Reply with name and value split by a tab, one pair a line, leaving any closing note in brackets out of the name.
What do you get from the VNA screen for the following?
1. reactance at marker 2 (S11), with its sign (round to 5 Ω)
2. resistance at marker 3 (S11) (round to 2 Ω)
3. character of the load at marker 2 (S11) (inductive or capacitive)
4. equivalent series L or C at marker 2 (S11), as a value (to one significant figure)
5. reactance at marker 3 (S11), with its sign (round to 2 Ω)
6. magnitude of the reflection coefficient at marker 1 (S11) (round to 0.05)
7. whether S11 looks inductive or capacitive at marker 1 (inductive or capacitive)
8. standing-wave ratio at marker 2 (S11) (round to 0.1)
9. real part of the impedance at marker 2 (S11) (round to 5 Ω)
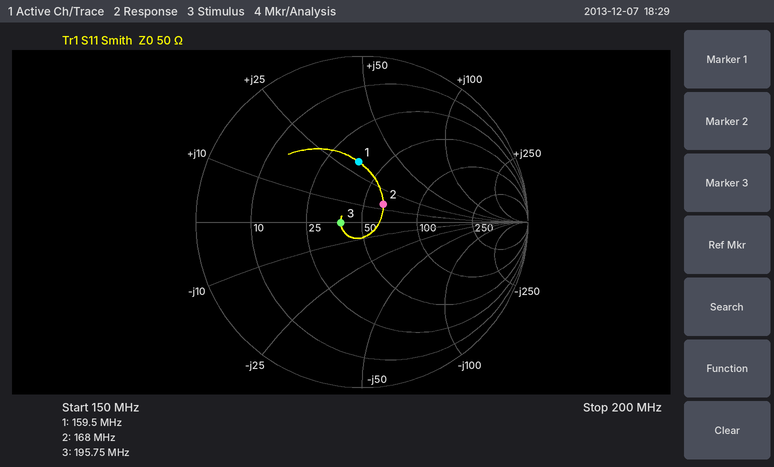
reactance at marker 2 (S11), with its sign	+15 Ω
resistance at marker 3 (S11)	38 Ω
character of the load at marker 2 (S11)	inductive
equivalent series L or C at marker 2 (S11), as a value	10 nH
reactance at marker 3 (S11), with its sign	0 Ω
magnitude of the reflection coefficient at marker 1 (S11)	0.35
whether S11 looks inductive or capacitive at marker 1	inductive
standing-wave ratio at marker 2 (S11)	1.4
real part of the impedance at marker 2 (S11)	65 Ω
